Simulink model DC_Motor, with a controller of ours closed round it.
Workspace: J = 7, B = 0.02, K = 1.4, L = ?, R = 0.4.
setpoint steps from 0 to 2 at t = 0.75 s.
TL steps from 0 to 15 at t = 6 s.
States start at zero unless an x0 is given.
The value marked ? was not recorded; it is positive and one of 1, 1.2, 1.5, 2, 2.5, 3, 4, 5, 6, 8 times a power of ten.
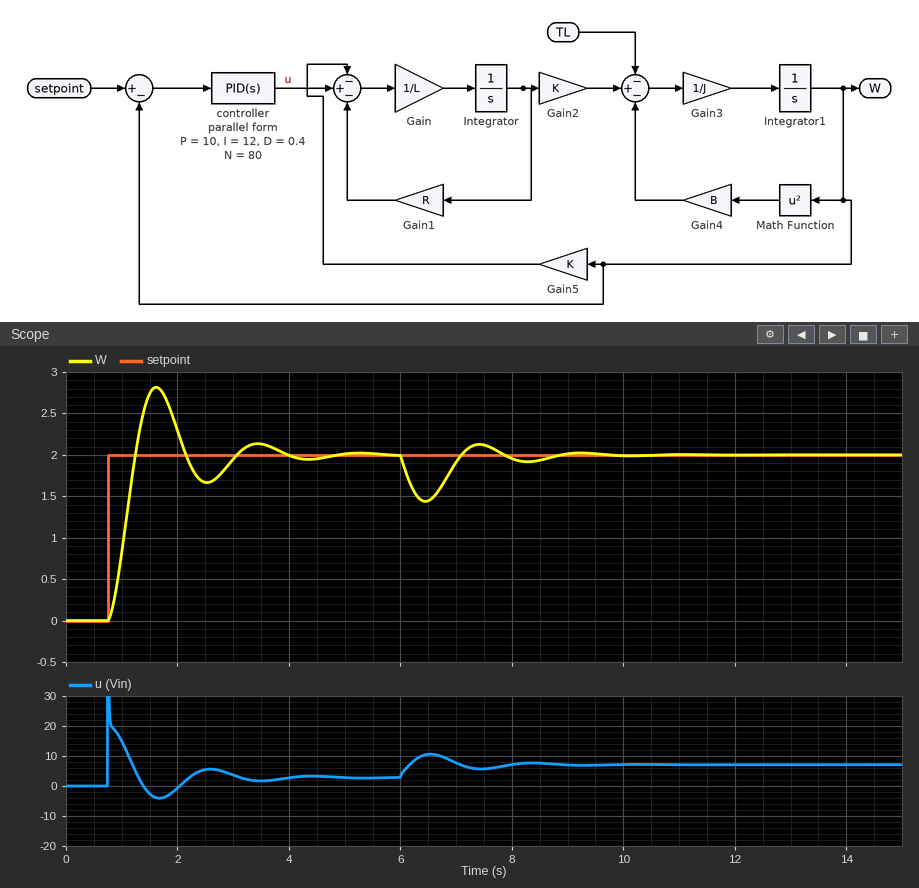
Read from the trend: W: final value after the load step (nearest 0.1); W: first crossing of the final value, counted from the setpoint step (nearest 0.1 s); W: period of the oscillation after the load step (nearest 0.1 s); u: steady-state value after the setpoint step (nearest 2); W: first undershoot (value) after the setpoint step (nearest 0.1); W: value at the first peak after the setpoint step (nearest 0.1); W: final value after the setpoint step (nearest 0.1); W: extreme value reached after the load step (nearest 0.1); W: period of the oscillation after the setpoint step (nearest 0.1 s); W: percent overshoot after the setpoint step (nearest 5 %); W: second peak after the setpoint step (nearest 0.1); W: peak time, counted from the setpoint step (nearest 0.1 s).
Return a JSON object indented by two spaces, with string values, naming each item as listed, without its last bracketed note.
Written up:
{
  "W: final value after the load step": "2.0",
  "W: first crossing of the final value, counted from the setpoint step": "0.5 s",
  "W: period of the oscillation after the load step": "1.8 s",
  "u: steady-state value after the setpoint step": "2",
  "W: first undershoot (value) after the setpoint step": "1.7",
  "W: value at the first peak after the setpoint step": "2.8",
  "W: final value after the setpoint step": "2.0",
  "W: extreme value reached after the load step": "1.4",
  "W: period of the oscillation after the setpoint step": "1.8 s",
  "W: percent overshoot after the setpoint step": "40 %",
  "W: second peak after the setpoint step": "2.1",
  "W: peak time, counted from the setpoint step": "0.9 s"
}
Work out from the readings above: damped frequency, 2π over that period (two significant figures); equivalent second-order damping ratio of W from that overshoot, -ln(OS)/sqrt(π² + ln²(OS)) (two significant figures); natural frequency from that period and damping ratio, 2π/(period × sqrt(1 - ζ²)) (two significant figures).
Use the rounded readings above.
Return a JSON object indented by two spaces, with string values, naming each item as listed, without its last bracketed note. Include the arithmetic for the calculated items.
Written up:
{
  "damped frequency, 2π over that period": "2π / 1.8 = 3.5 rad/s",
  "equivalent second-order damping ratio of W from that overshoot, -ln(OS)/sqrt(π² + ln²(OS))": "ln(0.4) = -0.916; 0.916 / sqrt(9.870 + 0.840) = 0.28",
  "natural frequency from that period and damping ratio, 2π/(period × sqrt(1 - ζ²))": "2π / (1.8 × sqrt(1 - 0.28²)) = 3.6 rad/s"
}
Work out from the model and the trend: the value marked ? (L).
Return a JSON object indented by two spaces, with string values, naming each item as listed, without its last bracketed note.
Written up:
{
  "the value marked ?": "0.15"
}
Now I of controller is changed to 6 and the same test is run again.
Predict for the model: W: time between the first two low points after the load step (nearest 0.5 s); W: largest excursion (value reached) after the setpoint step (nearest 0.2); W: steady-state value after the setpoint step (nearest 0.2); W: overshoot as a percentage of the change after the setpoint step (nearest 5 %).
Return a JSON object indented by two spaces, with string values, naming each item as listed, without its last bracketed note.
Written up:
{
  "W: time between the first two low points after the load step": "1.5 s",
  "W: largest excursion (value reached) after the setpoint step": "2.6",
  "W: steady-state value after the setpoint step": "2.0",
  "W: overshoot as a percentage of the change after the setpoint step": "25 %"
}
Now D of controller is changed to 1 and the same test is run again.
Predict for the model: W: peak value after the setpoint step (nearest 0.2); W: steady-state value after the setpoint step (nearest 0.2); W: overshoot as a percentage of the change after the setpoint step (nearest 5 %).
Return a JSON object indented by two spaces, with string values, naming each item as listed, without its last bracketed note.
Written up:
{
  "W: peak value after the setpoint step": "2.6",
  "W: steady-state value after the setpoint step": "2.0",
  "W: overshoot as a percentage of the change after the setpoint step": "30 %"
}
